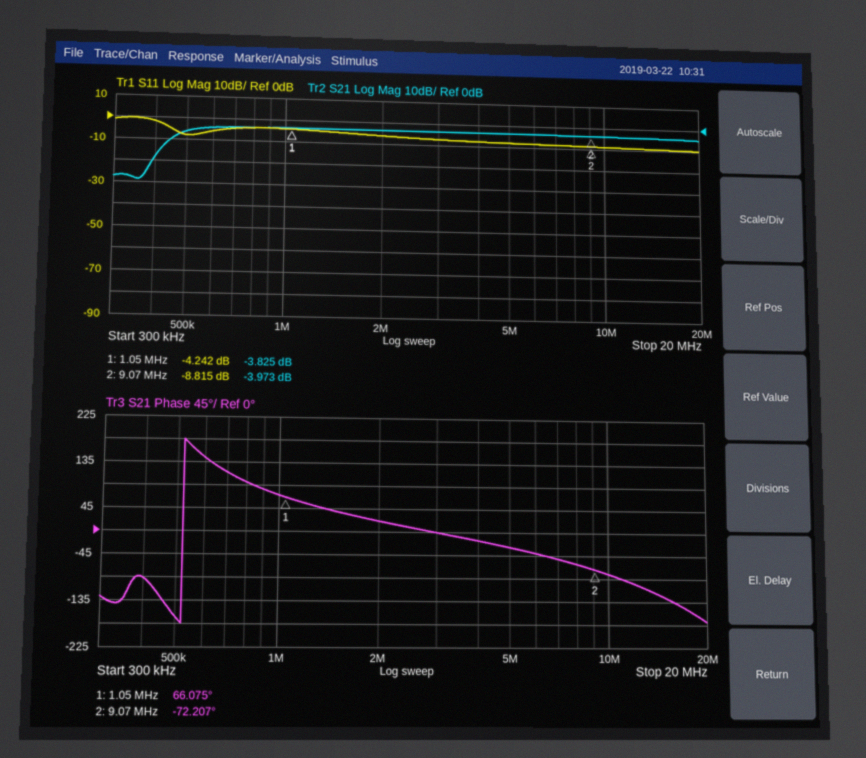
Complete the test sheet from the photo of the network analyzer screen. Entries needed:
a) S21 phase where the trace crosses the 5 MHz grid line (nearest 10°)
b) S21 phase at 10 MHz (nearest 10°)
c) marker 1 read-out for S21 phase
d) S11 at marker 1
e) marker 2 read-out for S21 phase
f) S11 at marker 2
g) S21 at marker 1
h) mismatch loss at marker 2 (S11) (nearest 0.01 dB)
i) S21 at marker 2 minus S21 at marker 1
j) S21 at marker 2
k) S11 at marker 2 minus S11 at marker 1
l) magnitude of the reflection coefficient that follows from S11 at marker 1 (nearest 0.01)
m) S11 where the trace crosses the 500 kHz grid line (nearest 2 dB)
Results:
-30°
-80°
66.075°
-4.242 dB
-72.207°
-8.815 dB
-3.825 dB
0.61 dB
-0.148 dB
-3.973 dB
-4.573 dB
0.61
-8 dB
